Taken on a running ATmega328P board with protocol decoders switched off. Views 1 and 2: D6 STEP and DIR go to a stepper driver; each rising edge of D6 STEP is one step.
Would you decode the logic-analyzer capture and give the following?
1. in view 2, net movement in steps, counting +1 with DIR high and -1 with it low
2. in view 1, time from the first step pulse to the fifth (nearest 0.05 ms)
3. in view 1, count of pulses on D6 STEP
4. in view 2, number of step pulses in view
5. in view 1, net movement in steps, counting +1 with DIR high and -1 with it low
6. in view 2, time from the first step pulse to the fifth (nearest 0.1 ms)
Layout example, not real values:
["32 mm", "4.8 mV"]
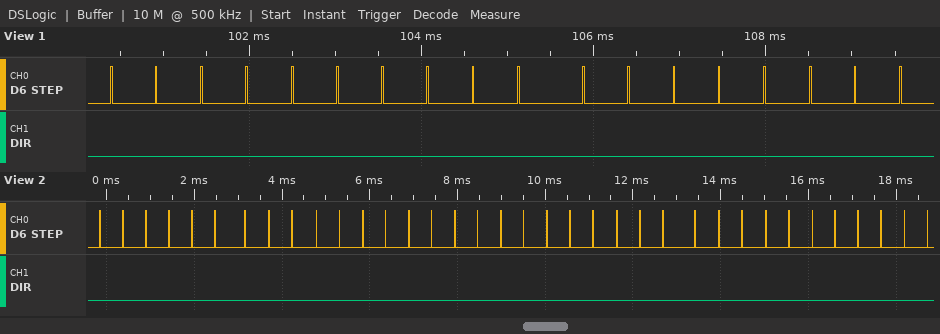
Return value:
["-36", "2.10 ms", "18", "36", "-18", "2.1 ms"]
